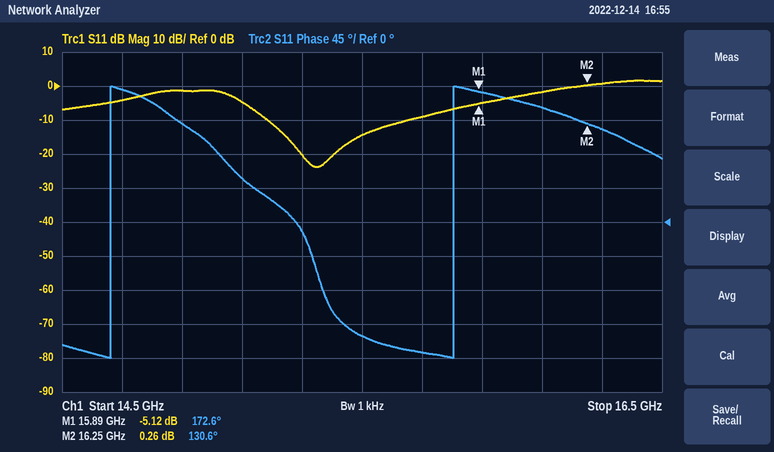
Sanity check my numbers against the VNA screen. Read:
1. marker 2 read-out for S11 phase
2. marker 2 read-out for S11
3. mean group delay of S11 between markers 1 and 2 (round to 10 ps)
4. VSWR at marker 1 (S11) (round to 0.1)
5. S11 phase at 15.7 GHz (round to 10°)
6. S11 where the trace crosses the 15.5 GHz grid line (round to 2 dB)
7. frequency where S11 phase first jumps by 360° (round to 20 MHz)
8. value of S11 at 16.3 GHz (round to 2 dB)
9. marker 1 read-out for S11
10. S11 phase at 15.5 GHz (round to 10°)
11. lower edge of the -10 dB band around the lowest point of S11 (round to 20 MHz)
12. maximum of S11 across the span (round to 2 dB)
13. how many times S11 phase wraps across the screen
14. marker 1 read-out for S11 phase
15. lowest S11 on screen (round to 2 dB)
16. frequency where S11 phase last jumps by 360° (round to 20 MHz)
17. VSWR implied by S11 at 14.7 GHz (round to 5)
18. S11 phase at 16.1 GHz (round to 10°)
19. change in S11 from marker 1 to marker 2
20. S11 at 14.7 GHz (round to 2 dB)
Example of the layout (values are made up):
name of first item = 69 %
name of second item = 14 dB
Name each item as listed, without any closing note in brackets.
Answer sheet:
marker 2 read-out for S11 phase = 130.6°
marker 2 read-out for S11 = 0.26 dB
mean group delay of S11 between markers 1 and 2 = 320 ps
VSWR at marker 1 (S11) = 3.5
S11 phase at 15.7 GHz = -170°
S11 where the trace crosses the 15.5 GHz grid line = -14 dB
frequency where S11 phase first jumps by 360° = 14.66 GHz
value of S11 at 16.3 GHz = 0 dB
marker 1 read-out for S11 = -5.12 dB
S11 phase at 15.5 GHz = -150°
lower edge of the -10 dB band around the lowest point of S11 = 15.18 GHz
maximum of S11 across the span = 2 dB
how many times S11 phase wraps across the screen = 2
marker 1 read-out for S11 phase = 172.6°
lowest S11 on screen = -24 dB
frequency where S11 phase last jumps by 360° = 15.80 GHz
VSWR implied by S11 at 14.7 GHz = 5
S11 phase at 16.1 GHz = 150°
change in S11 from marker 1 to marker 2 = 5.38 dB
S11 at 14.7 GHz = -4 dB
